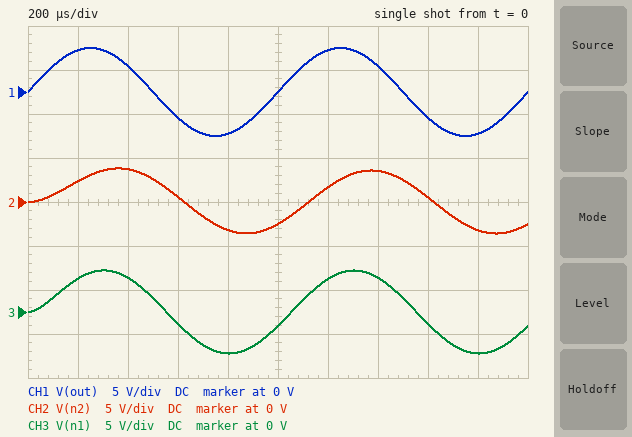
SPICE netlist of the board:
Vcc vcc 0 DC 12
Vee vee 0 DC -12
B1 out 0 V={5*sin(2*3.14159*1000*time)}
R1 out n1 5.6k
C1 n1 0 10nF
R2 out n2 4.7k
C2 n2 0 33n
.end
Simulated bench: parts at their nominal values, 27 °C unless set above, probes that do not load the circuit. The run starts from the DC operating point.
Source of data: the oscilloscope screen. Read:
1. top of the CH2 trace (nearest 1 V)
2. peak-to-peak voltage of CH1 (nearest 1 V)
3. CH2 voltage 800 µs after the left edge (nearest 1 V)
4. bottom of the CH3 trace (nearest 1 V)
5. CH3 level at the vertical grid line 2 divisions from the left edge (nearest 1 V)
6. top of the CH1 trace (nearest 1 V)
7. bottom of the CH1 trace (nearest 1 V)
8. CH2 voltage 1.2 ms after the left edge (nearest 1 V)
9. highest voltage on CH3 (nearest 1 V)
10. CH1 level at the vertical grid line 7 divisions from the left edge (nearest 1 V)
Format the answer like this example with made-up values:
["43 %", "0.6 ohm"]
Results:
["4 V", "10 V", "-3 V", "-5 V", "4 V", "5 V", "-5 V", "2 V", "5 V", "3 V"]
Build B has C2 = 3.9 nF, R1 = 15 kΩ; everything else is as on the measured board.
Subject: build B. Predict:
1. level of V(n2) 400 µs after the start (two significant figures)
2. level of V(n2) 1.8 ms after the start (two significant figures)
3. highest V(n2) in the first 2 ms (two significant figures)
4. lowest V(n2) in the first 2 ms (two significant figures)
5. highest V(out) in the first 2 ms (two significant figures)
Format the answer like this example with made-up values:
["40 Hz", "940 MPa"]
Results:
["3.4 V", "-4.9 V", "5.0 V", "-5.0 V", "5.0 V"]
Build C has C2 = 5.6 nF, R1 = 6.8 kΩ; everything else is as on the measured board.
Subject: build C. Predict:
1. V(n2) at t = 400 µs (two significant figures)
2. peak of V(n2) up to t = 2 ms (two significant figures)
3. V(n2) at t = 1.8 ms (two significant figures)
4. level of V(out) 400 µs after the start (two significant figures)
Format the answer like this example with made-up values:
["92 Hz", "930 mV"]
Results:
["3.5 V", "4.9 V", "-4.9 V", "2.9 V"]
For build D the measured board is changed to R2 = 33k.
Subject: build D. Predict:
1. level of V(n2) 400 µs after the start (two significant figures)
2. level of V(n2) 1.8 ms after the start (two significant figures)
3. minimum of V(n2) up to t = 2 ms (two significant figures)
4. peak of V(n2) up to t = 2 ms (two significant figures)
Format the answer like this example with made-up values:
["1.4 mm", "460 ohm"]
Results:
["1.1 V", "-180 mV", "-610 mV", "1.2 V"]
